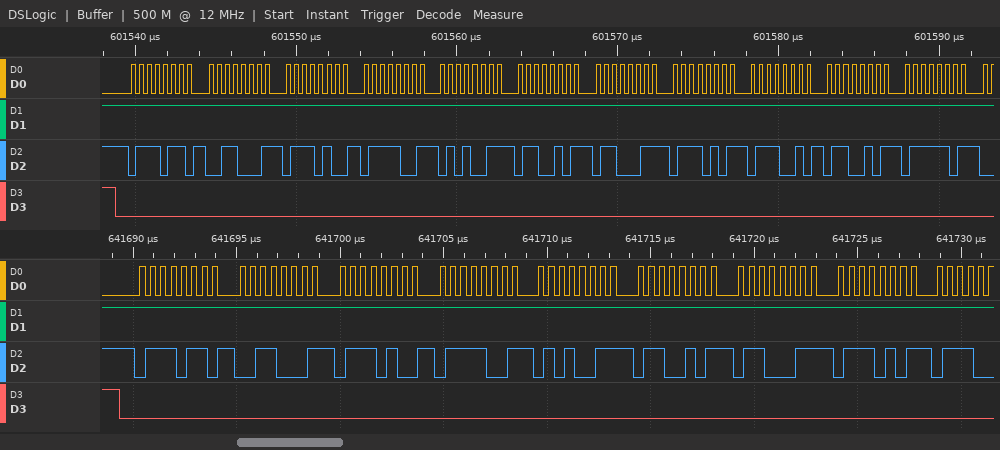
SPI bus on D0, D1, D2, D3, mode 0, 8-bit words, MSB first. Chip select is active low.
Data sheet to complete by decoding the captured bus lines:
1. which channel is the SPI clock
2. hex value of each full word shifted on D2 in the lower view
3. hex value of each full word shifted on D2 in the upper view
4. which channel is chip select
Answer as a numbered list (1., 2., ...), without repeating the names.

1. D0
2. 76, 31, 74, 79, 53, 65, 63, 75
3. 76, 31, 74, 79, 53, 65, 63, 75, 72, 65, 7D
4. D3
